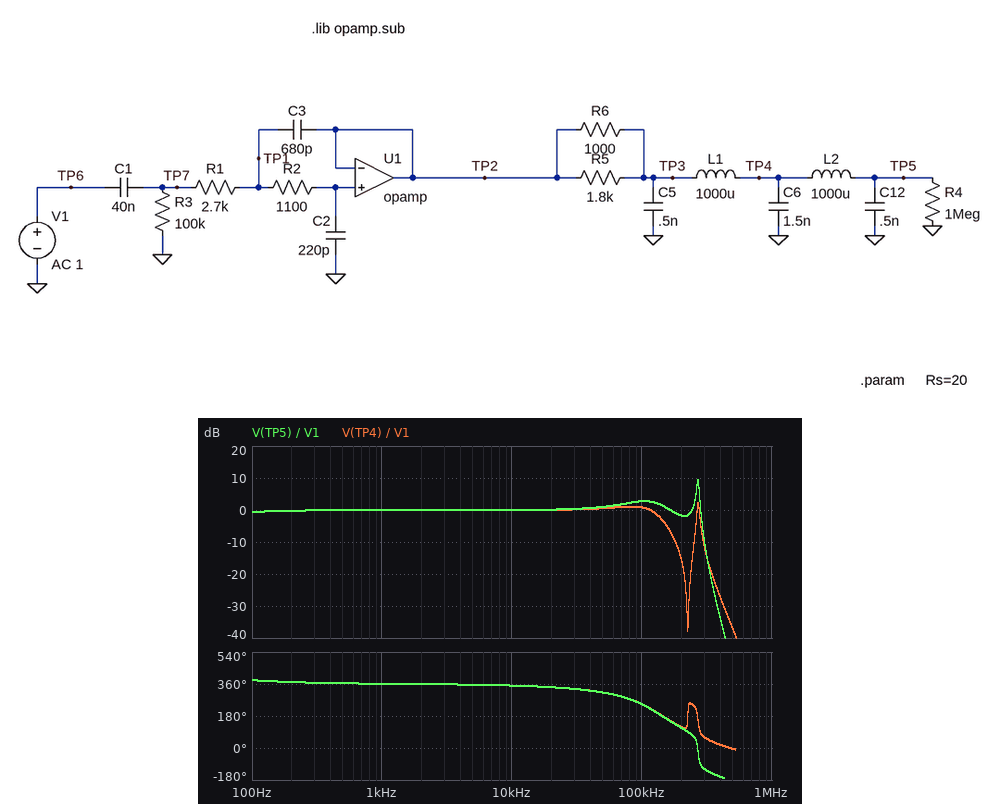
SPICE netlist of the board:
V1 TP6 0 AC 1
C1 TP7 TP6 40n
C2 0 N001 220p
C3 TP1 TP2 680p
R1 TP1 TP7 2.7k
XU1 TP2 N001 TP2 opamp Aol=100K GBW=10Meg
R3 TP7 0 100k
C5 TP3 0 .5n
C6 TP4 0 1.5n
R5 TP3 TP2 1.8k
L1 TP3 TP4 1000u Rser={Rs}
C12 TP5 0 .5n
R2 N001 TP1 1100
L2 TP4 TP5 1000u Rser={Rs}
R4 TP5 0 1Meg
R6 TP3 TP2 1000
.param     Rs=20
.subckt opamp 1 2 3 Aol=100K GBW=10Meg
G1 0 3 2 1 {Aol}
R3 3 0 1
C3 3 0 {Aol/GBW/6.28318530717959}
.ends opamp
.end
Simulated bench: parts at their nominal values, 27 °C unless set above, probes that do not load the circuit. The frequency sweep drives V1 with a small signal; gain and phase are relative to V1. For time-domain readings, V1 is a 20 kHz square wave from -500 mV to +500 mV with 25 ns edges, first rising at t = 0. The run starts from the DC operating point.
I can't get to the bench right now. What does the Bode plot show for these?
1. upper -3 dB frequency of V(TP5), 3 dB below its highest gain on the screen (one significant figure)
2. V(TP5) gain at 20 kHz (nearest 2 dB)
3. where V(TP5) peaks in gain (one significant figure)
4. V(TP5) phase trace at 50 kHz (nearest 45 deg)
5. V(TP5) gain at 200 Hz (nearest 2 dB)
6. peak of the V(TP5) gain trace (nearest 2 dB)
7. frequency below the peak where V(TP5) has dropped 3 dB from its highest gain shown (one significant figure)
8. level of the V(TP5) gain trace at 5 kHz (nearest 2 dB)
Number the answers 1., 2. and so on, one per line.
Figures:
1. 300 kHz
2. 0 dB
3. 300 kHz
4. 315 deg
5. 0 dB
6. 10 dB
7. 300 kHz
8. 0 dB
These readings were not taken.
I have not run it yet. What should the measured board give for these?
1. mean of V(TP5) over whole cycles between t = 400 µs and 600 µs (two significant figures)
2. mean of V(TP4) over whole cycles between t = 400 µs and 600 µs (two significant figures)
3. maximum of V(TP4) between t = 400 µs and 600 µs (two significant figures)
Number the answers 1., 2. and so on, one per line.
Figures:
1. 440 mV
2. 440 mV
3. 1.2 V
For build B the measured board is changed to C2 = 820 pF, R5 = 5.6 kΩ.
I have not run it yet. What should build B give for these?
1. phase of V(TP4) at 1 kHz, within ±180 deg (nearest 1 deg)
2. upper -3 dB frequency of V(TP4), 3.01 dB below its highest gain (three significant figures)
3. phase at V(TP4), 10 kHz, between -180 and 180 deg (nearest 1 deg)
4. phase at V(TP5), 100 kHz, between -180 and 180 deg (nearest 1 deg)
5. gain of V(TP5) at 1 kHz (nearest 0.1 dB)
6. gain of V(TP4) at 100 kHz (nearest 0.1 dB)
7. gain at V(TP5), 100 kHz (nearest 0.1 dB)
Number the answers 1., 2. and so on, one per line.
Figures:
1. 0 deg
2. 56.8 kHz
3. -19 deg
4. -163 deg
5. -0.2 dB
6. -7.7 dB
7. -5.8 dB
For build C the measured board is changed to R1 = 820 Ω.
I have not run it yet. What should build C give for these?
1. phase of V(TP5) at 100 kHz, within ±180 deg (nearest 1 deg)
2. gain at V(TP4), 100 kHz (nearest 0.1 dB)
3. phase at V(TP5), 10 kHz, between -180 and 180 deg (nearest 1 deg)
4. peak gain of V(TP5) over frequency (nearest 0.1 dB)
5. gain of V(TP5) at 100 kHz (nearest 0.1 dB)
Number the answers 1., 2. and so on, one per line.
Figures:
1. -97 deg
2. 0.7 dB
3. -7 deg
4. 13.3 dB
5. 2.6 dB
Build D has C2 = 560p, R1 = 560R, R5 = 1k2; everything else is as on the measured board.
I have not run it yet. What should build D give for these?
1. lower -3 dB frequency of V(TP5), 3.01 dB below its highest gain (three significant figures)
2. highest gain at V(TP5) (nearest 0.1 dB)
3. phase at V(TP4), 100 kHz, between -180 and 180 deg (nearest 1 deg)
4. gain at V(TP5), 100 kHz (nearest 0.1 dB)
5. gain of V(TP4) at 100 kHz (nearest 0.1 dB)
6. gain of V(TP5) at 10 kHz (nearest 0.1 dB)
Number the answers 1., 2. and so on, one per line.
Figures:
1. 264 kHz
2. 9.5 dB
3. -112 deg
4. 3.1 dB
5. 1.2 dB
6. -0.1 dB
